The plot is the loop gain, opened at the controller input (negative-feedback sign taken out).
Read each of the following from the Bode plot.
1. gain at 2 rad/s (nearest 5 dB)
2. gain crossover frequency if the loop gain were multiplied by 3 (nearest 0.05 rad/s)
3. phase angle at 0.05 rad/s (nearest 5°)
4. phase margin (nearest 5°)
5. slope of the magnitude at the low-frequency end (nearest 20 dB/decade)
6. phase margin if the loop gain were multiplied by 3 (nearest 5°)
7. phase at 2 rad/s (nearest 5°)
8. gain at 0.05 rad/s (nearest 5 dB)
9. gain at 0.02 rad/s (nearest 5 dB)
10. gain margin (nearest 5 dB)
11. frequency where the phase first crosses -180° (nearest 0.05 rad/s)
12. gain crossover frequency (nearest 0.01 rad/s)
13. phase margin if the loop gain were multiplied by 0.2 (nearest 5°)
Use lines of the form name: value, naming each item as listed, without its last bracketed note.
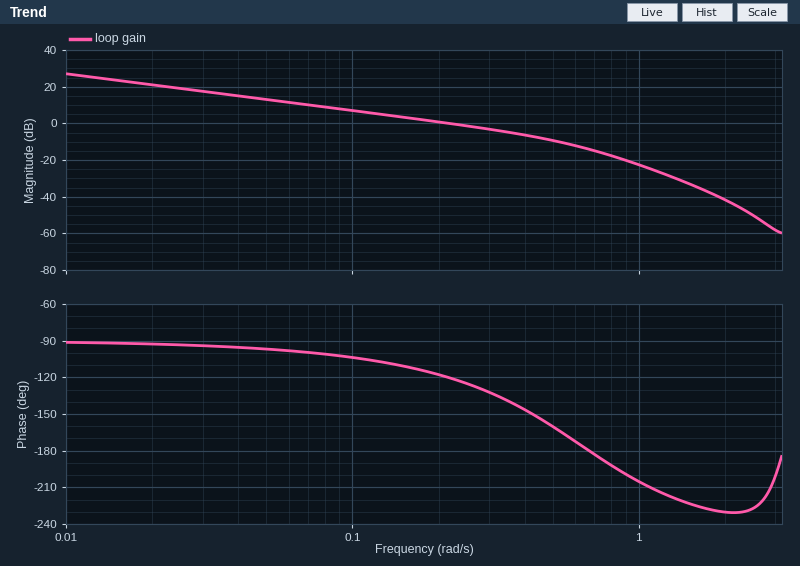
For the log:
gain at 2 rad/s: -40 dB
gain crossover frequency if the loop gain were multiplied by 3: 0.50 rad/s
phase angle at 0.05 rad/s: -95°
phase margin: 60°
slope of the magnitude at the low-frequency end: -20 dB/decade
phase margin if the loop gain were multiplied by 3: 20°
phase at 2 rad/s: -230°
gain at 0.05 rad/s: 15 dB
gain at 0.02 rad/s: 20 dB
gain margin: 15 dB
frequency where the phase first crosses -180°: 0.65 rad/s
gain crossover frequency: 0.22 rad/s
phase margin if the loop gain were multiplied by 0.2: 85°
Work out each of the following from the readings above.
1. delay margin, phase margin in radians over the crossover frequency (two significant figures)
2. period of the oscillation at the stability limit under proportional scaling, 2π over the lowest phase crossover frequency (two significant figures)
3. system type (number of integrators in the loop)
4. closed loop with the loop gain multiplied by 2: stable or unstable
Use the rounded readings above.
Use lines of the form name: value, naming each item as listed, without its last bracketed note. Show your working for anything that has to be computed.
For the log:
delay margin, phase margin in radians over the crossover frequency: 60 × π / 180 / 0.22 = 4.8 s
period of the oscillation at the stability limit under proportional scaling, 2π over the lowest phase crossover frequency: 2π / 0.65 = 9.7 s
system type: 1
closed loop with the loop gain multiplied by 2: stable or unstable: stable
